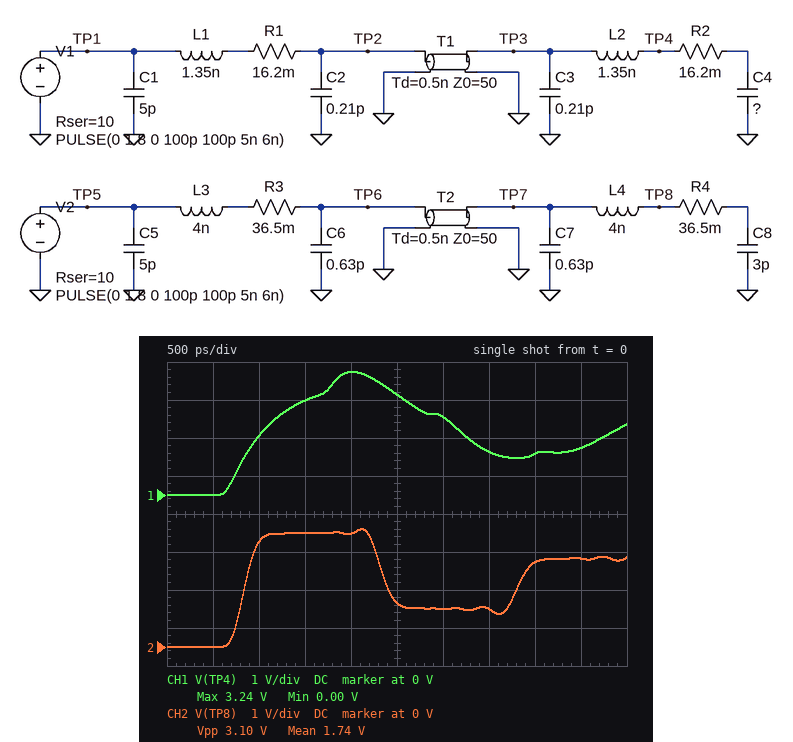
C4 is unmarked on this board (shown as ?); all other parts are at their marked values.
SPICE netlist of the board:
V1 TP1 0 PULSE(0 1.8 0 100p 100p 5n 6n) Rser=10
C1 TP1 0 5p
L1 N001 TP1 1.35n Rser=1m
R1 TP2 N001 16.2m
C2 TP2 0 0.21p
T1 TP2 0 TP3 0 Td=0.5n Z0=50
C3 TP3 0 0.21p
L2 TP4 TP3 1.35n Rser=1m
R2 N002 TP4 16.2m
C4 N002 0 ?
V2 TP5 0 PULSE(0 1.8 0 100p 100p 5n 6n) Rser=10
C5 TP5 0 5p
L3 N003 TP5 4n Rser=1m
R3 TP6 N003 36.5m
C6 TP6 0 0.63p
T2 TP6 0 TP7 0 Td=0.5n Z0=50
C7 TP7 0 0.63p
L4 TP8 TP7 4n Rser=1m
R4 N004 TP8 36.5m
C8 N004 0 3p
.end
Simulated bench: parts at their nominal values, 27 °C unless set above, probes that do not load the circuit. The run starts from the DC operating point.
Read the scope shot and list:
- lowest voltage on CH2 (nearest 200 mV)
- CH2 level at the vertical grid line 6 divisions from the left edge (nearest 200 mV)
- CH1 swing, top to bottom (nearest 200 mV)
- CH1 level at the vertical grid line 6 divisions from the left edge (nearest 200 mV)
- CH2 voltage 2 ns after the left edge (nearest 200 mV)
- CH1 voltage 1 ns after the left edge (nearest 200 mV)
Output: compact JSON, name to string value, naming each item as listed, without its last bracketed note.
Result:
{"lowest voltage on CH2": "0 V", "CH2 level at the vertical grid line 6 divisions from the left edge": "1.0 V", "CH1 swing, top to bottom": "3.2 V", "CH1 level at the vertical grid line 6 divisions from the left edge": "2.0 V", "CH2 voltage 2 ns after the left edge": "3.0 V", "CH1 voltage 1 ns after the left edge": "1.6 V"}
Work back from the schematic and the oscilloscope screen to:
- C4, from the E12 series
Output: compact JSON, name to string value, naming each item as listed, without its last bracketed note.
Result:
{"C4, from the E12 series": "10 pF"}
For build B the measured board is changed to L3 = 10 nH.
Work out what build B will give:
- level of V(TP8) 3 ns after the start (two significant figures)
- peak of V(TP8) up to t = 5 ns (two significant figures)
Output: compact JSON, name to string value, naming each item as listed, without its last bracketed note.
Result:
{"level of V(TP8) 3 ns after the start": "1.1 V", "peak of V(TP8) up to t = 5 ns": "3.4 V"}
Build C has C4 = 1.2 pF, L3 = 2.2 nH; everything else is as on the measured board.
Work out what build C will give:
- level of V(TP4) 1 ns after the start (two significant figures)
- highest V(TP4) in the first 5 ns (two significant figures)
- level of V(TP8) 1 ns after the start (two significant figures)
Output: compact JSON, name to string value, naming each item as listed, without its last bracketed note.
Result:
{"level of V(TP4) 1 ns after the start": "3.0 V", "highest V(TP4) in the first 5 ns": "3.1 V", "level of V(TP8) 1 ns after the start": "2.9 V"}
